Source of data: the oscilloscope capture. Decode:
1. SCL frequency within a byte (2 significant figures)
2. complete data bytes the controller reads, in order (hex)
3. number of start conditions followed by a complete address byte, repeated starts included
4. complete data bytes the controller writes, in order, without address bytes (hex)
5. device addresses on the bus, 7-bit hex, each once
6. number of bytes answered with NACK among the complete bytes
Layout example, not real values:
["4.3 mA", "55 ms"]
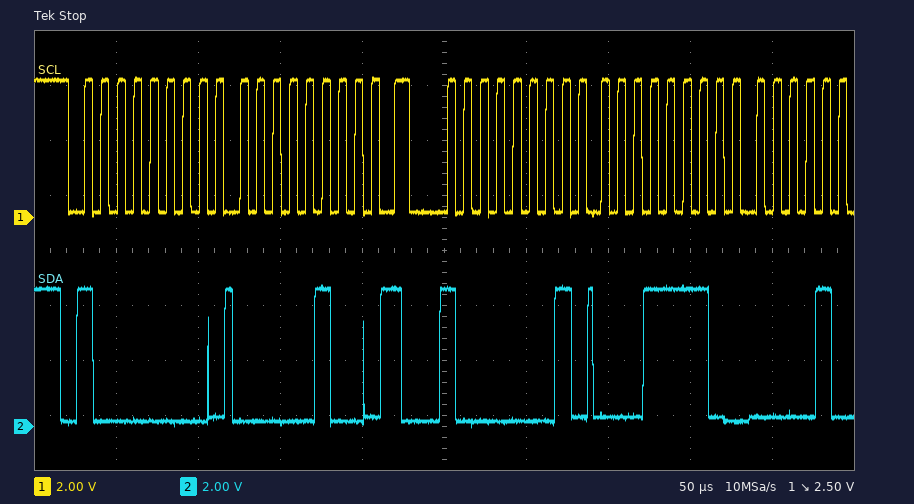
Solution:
["100 kHz", "1E", "2", "04", "0x40", "0"]
